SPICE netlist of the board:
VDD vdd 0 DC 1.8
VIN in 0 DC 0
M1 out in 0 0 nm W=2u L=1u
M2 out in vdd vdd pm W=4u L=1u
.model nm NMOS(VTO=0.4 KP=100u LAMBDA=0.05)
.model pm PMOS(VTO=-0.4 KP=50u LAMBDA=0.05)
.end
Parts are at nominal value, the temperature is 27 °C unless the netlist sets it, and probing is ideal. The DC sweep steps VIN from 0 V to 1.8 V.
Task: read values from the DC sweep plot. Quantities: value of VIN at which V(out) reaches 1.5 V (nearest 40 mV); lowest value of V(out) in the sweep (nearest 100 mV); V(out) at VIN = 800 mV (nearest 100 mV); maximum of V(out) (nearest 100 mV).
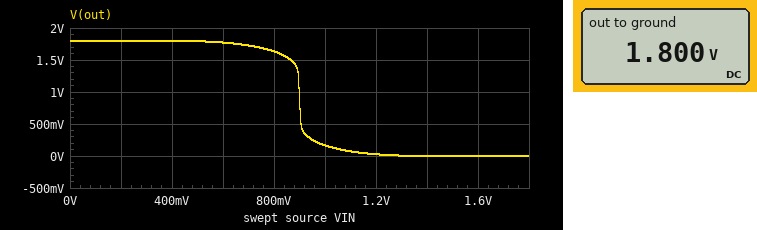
880 mV
0 V
1.6 V
1.8 V
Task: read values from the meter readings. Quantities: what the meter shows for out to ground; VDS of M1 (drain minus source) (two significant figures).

1.800 V
1.8 V
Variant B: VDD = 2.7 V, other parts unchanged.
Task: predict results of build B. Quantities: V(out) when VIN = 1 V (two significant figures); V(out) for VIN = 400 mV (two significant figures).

2.5 V
2.7 V
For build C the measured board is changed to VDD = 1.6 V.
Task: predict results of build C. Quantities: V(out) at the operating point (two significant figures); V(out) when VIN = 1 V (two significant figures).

1.6 V
37 mV
